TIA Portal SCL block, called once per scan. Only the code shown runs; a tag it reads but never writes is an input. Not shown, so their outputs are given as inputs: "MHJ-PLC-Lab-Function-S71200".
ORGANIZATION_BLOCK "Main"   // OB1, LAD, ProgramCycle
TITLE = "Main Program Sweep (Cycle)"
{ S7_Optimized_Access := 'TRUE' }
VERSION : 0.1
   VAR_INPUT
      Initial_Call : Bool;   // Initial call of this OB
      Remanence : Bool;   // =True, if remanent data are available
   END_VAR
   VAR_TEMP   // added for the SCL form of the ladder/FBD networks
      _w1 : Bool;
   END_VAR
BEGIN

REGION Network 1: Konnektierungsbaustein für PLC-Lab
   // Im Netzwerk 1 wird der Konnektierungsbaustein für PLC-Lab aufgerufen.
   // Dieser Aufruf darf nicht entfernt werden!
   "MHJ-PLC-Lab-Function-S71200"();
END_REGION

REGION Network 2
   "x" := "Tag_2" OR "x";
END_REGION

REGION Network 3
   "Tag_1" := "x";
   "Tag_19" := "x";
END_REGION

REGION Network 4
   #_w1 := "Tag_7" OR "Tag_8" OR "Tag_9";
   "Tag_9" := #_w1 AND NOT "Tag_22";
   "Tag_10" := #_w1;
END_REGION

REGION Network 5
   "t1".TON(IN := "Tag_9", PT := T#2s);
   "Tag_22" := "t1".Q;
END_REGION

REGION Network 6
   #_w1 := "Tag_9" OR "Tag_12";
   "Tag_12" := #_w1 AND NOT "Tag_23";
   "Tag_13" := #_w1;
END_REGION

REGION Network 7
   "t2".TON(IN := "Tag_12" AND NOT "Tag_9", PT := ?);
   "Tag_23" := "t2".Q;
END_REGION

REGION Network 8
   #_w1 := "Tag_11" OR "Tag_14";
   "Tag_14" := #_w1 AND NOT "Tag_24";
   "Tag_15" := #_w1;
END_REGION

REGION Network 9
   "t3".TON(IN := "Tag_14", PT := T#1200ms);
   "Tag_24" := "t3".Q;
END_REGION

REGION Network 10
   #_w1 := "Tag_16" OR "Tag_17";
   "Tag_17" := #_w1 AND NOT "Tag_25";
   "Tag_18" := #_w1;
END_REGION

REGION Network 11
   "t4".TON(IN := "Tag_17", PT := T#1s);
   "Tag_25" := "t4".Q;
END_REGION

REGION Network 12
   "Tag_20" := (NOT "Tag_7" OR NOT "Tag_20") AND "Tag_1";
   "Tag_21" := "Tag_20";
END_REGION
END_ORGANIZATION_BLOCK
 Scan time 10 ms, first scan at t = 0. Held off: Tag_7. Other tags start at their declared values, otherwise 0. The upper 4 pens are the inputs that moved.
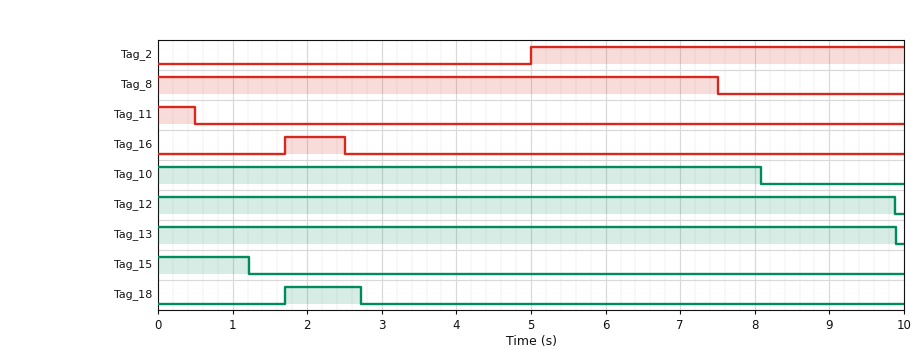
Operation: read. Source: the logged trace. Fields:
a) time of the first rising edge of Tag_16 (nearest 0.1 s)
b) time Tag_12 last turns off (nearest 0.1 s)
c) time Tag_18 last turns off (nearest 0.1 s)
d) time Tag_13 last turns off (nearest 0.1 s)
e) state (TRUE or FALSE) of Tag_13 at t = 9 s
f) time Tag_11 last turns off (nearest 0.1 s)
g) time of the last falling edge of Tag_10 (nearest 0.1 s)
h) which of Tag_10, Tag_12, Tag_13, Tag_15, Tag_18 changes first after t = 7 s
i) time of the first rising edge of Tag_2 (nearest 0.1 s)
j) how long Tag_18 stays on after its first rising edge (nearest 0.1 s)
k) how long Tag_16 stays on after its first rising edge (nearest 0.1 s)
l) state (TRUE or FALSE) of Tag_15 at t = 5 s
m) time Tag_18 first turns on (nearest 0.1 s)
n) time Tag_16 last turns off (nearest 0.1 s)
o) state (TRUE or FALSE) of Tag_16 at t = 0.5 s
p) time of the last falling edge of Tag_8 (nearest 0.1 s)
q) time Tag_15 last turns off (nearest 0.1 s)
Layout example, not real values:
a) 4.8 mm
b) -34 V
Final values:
a) 1.7 s
b) 9.9 s
c) 2.7 s
d) 9.9 s
e) TRUE
f) 0.5 s
g) 8.1 s
h) Tag_10
i) 5.0 s
j) 1.0 s
k) 0.8 s
l) FALSE
m) 1.7 s
n) 2.5 s
o) FALSE
p) 7.5 s
q) 1.2 s
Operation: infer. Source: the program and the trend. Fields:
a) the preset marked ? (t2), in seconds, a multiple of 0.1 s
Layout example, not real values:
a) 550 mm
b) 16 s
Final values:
a) 1.8 s
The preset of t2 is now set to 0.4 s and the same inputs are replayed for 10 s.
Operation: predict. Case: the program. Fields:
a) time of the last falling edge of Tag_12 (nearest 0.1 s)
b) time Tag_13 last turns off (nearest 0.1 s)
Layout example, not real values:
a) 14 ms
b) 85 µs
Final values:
a) 8.5 s
b) 8.5 s
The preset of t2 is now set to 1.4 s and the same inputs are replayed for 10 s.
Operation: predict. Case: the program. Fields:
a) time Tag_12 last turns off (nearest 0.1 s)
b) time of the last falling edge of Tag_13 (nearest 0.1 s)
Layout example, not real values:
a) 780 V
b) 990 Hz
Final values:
a) 9.5 s
b) 9.5 s
